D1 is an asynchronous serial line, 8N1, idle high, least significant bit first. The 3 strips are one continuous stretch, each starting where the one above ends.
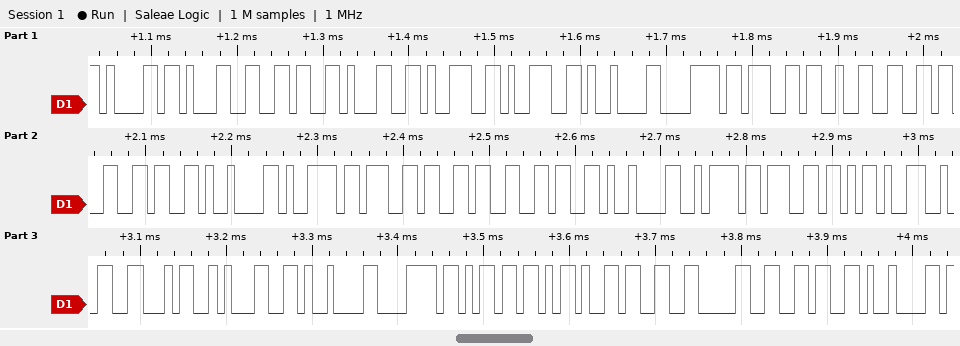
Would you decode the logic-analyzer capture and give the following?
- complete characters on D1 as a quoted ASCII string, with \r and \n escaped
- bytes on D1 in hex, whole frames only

"a16199\txg266\tyg66\tzg-241\txm-306\t"
0x61 0x31 0x36 0x31 0x39 0x39 0x09 0x78 0x67 0x32 0x36 0x36 0x09 0x79 0x67 0x36 0x36 0x09 0x7A 0x67 0x2D 0x32 0x34 0x31 0x09 0x78 0x6D 0x2D 0x33 0x30 0x36 0x09
